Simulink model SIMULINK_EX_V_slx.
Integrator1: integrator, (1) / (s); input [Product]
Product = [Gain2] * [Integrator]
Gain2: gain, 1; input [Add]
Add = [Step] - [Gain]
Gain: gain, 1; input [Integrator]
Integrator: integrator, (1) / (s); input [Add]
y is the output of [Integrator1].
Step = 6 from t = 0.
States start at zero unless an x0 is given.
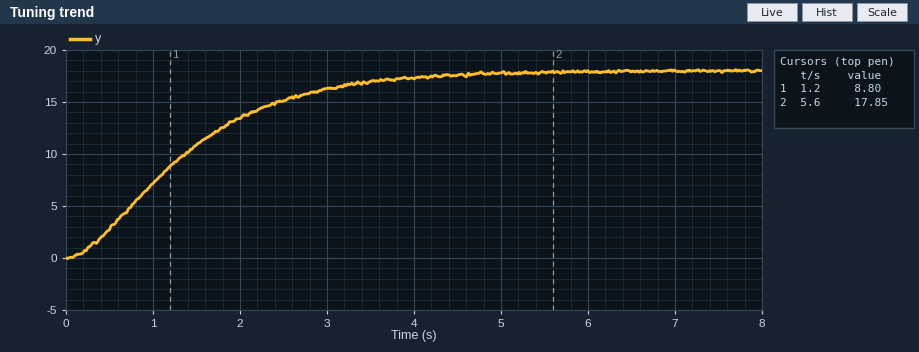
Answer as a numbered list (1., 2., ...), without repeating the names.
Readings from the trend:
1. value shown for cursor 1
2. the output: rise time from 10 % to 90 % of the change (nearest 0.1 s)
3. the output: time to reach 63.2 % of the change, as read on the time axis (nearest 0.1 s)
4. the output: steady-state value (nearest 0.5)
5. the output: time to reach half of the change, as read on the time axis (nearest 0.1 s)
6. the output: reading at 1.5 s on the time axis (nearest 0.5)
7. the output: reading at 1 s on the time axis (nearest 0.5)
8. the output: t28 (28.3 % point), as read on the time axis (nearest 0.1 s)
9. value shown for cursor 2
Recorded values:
1. 8.80
2. 2.6 s
3. 1.6 s
4. 18.0
5. 1.2 s
6. 11.0
7. 7.0
8. 0.8 s
9. 17.85
